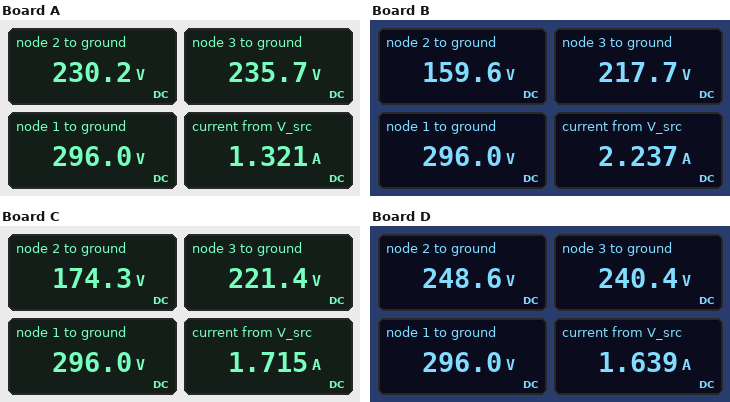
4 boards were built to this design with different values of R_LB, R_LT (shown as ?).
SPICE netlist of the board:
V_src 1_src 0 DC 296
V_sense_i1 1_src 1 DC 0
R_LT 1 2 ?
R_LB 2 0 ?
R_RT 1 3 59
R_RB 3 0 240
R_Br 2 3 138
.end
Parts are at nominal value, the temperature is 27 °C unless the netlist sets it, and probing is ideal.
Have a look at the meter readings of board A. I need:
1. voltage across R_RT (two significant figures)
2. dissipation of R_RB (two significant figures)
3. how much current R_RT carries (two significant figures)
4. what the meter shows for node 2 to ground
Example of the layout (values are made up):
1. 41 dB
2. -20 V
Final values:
1. 60 V
2. 230 W
3. 1.0 A
4. 230.2 V
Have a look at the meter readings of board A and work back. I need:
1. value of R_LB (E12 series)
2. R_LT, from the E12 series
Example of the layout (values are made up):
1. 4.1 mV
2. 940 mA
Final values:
1. 680 Ω
2. 220 Ω
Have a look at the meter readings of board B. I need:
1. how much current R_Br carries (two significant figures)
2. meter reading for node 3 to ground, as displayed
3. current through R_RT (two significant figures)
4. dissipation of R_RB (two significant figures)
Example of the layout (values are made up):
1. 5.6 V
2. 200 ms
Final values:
1. 420 mA
2. 217.7 V
3. 1.3 A
4. 200 W
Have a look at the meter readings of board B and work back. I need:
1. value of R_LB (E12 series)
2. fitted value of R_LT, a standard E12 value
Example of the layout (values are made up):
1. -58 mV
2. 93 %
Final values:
1. 120 Ω
2. 150 Ω
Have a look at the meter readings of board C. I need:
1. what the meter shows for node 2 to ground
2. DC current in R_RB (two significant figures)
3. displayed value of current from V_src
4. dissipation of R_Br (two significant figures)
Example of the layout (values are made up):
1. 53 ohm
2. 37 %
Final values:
1. 174.3 V
2. 920 mA
3. 1.715 A
4. 16 W
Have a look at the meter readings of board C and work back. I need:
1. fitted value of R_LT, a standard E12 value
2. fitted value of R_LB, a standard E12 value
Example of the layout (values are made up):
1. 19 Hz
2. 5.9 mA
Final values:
1. 270 Ω
2. 220 Ω
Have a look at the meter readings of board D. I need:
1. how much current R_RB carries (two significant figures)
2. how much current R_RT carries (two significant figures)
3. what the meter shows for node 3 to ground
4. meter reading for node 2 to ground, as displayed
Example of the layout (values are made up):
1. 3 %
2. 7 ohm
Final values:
1. 1.0 A
2. 940 mA
3. 240.4 V
4. 248.6 V
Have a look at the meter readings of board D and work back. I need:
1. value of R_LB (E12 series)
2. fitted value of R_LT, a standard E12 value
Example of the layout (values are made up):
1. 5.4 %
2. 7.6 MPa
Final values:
1. 390 Ω
2. 68 Ω
